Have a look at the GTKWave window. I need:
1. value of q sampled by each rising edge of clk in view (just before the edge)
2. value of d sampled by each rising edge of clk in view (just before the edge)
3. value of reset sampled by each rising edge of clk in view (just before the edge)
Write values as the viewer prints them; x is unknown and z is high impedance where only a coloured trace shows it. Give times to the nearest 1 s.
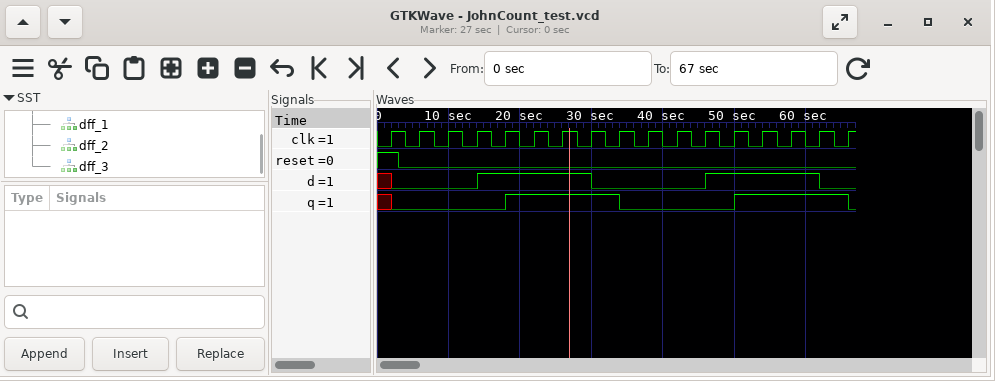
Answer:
x 0 0 0 0 1 1 1 1 0 0 0 0 1 1 1 1
x 0 0 0 1 1 1 1 0 0 0 0 1 1 1 1 0
1 0 0 0 0 0 0 0 0 0 0 0 0 0 0 0 0
